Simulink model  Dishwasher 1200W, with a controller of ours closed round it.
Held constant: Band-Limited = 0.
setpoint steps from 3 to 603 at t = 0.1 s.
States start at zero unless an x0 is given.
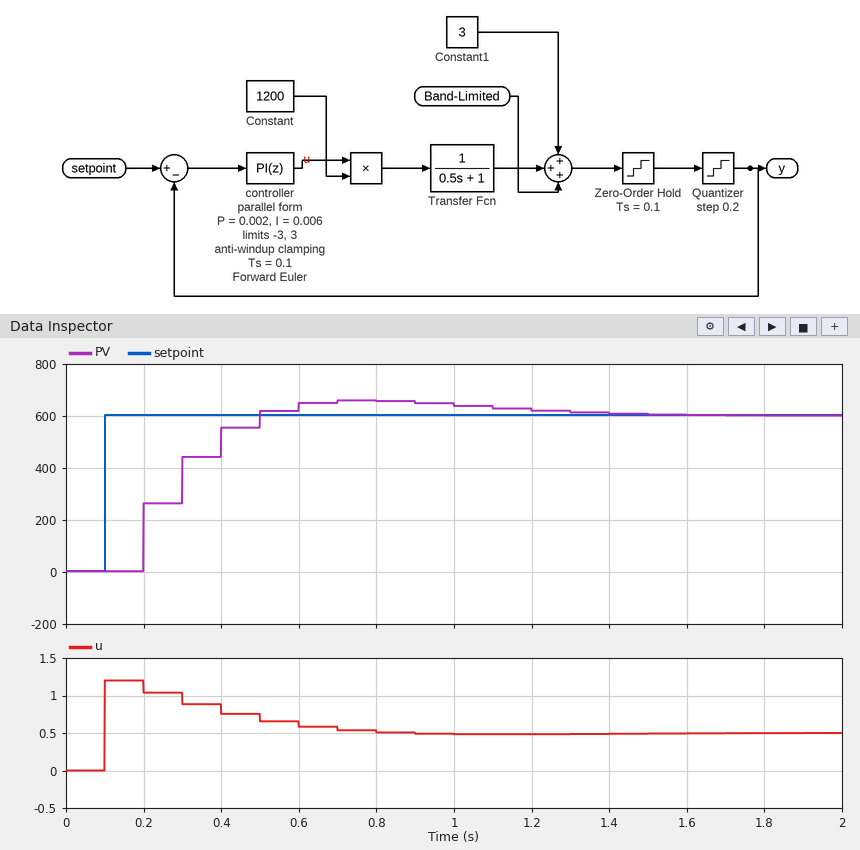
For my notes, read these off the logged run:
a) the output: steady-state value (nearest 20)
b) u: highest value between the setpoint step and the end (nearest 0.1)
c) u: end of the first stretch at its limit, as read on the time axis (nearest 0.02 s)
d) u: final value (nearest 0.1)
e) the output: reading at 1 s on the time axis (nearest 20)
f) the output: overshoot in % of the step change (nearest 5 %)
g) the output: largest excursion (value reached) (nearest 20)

600
1.2
0.20 s
0.5
640
10 %
660
